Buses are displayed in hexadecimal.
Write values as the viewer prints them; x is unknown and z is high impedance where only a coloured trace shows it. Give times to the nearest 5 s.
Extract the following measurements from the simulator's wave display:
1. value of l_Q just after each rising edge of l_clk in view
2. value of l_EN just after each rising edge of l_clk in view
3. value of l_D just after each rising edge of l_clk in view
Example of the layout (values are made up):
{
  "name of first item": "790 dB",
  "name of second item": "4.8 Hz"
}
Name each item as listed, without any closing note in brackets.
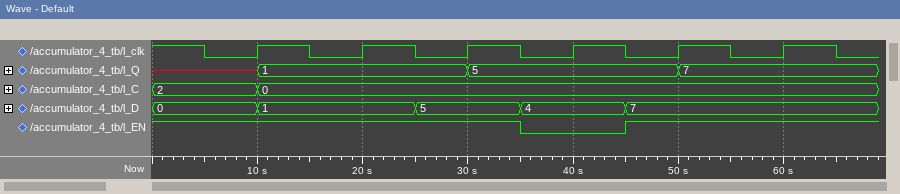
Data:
{
  "value of l_Q just after each rising edge of l_clk in view": "1, 1, 5, 5, 7, 7",
  "value of l_EN just after each rising edge of l_clk in view": "1 1 1 0 1 1",
  "value of l_D just after each rising edge of l_clk in view": "1, 1, 5, 4, 7, 7"
}
